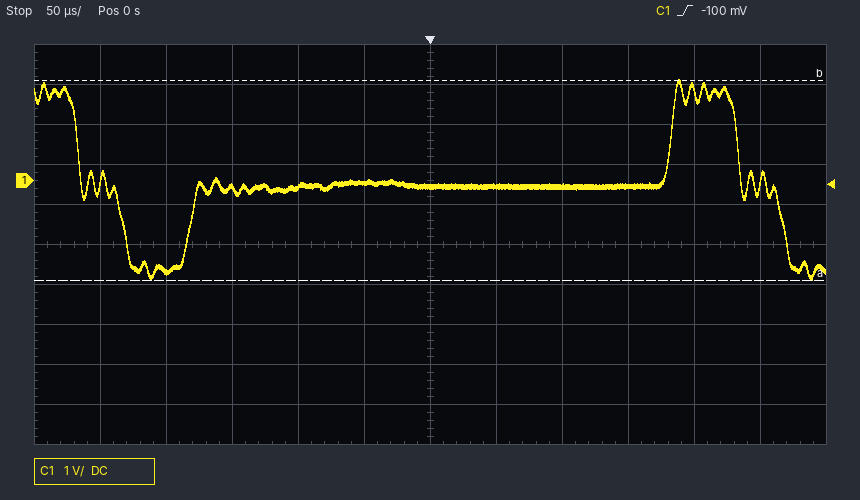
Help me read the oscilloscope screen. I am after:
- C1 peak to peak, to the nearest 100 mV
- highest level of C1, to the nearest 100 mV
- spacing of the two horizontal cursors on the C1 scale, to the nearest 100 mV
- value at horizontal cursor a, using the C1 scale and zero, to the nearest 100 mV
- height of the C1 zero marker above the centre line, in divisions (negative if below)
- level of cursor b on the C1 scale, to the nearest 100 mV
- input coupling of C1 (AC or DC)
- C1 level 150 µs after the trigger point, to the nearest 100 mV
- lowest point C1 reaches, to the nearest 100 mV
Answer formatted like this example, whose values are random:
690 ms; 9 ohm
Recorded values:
5.0 V; 2.5 V; 5.0 V; -2.5 V; +1.6 div; 2.5 V; DC; -100 mV; -2.5 V
